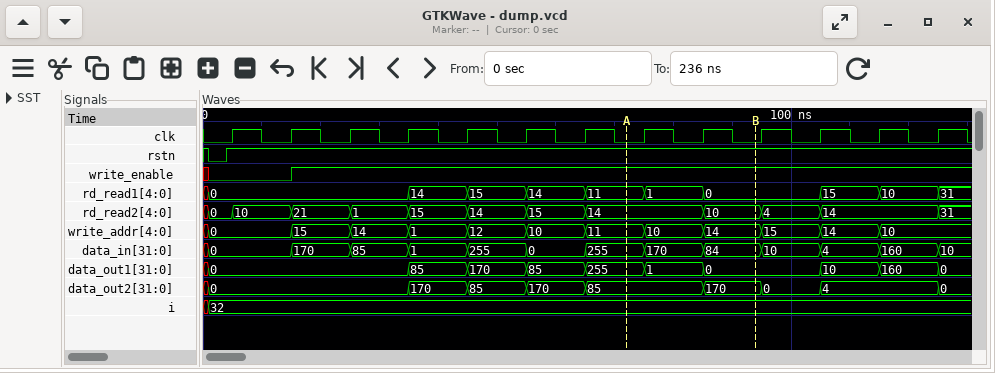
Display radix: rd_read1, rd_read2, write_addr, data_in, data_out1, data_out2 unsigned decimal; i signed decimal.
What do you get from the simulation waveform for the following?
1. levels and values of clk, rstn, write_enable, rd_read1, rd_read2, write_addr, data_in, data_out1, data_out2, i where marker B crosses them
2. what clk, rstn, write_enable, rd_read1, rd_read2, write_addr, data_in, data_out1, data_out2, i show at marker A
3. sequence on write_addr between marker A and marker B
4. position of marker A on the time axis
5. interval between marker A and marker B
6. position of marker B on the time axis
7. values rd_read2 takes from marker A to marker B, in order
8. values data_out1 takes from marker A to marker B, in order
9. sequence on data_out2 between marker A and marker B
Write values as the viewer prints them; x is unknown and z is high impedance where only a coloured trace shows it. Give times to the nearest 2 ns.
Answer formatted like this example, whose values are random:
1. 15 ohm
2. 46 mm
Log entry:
1. clk=0, rstn=1, write_enable=1, rd_read1=0, rd_read2=10, write_addr=14, data_in=84, data_out1=0, data_out2=170, i=32
2. clk=0, rstn=1, write_enable=1, rd_read1=11, rd_read2=14, write_addr=11, data_in=255, data_out1=255, data_out2=85, i=32
3. 11, 10, 14
4. 72 ns
5. 22 ns
6. 94 ns
7. 14, 10
8. 255, 1, 0
9. 85, 170
